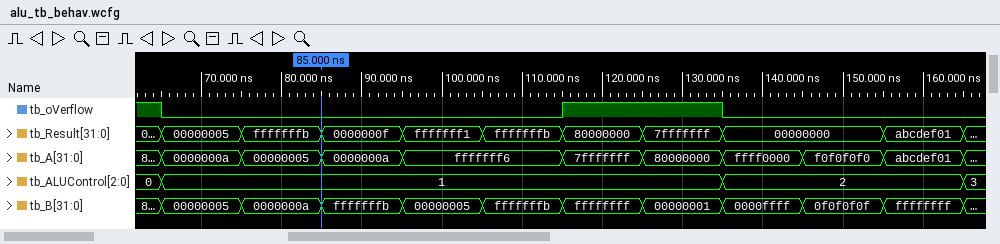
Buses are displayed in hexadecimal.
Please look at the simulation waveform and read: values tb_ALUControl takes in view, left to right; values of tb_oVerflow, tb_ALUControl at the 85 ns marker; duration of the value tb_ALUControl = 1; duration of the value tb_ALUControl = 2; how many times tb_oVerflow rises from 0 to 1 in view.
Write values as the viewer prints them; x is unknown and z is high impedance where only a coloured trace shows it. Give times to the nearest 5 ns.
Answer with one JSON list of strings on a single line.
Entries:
["0, 1, 2, 3", "tb_oVerflow=0, tb_ALUControl=1", "70 ns", "30 ns", "1"]
